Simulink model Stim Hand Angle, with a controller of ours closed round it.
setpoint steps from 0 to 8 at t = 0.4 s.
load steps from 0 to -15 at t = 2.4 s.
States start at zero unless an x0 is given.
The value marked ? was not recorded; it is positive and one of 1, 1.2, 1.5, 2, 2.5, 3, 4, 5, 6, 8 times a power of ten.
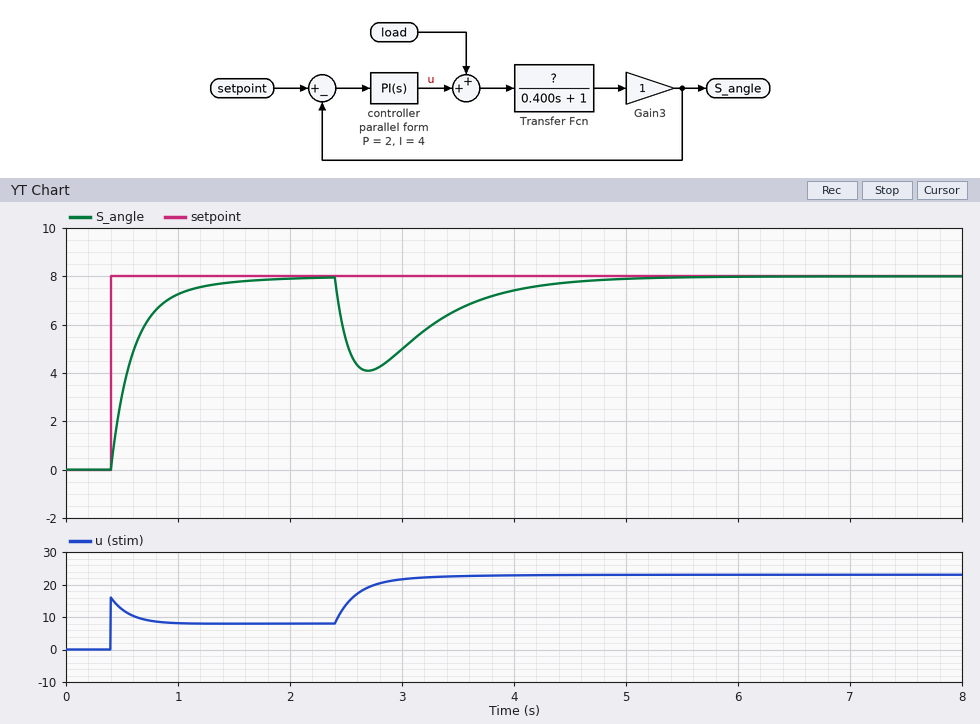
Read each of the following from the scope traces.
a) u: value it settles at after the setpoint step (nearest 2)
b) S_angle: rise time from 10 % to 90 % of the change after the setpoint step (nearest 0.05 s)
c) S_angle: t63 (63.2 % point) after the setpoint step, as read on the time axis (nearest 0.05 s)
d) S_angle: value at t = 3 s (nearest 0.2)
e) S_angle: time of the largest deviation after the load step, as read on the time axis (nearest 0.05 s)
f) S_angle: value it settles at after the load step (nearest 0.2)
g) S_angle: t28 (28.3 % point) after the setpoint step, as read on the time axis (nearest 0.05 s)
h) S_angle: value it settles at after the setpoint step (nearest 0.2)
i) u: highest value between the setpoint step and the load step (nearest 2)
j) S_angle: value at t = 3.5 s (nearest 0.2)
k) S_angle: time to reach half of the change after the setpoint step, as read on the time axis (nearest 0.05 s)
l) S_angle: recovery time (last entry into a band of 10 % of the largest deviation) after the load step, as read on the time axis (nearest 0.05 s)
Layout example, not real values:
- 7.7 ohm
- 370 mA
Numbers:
- 8
- 0.55 s
- 0.60 s
- 5.0
- 2.70 s
- 8.0
- 0.45 s
- 8.0
- 16
- 6.6
- 0.55 s
- 4.25 s
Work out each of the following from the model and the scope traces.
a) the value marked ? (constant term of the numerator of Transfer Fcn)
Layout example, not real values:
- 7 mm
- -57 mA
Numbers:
- 1
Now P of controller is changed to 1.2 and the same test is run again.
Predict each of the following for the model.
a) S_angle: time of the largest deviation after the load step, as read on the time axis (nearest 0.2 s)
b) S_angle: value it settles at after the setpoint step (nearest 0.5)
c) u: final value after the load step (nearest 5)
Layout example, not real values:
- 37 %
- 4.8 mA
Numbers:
- 2.8 s
- 8.0
- 25
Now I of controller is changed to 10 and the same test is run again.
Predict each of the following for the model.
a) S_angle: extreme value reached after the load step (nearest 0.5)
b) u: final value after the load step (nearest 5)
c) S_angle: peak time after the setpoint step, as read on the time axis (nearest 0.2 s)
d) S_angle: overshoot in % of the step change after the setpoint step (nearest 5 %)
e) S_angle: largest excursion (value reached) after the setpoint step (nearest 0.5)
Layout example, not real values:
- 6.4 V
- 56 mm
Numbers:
- 4.5
- 25
- 1.0 s
- 10 %
- 8.5
